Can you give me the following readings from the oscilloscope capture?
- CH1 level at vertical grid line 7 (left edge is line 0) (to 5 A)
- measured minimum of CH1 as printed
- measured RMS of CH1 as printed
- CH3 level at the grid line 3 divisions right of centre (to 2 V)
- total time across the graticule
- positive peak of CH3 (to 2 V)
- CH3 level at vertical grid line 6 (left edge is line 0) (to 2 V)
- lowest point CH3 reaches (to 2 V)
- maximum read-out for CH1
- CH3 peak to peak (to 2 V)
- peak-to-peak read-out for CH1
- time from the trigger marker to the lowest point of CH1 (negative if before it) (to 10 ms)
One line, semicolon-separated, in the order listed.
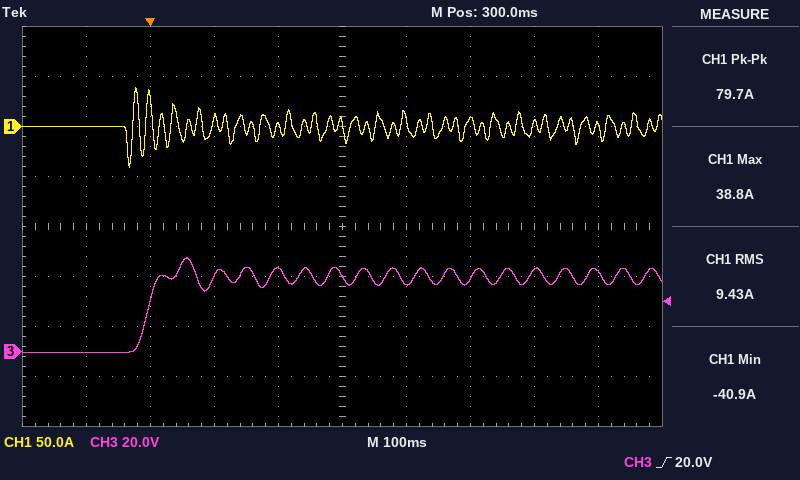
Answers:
5 A; -40.9 A; 9.43 A; 32 V; 1 s; 38 V; 28 V; 0 V; 38.8 A; 38 V; 79.7 A; -30 ms
